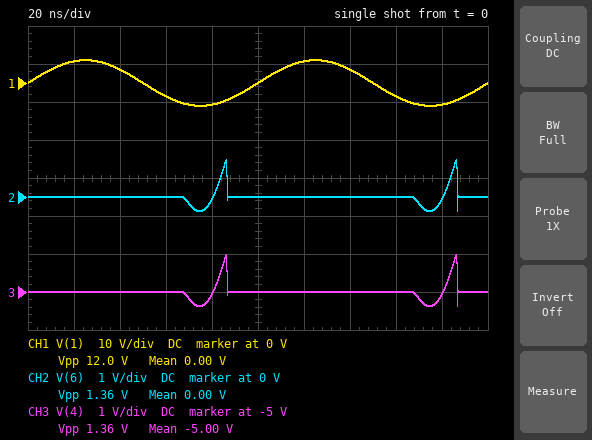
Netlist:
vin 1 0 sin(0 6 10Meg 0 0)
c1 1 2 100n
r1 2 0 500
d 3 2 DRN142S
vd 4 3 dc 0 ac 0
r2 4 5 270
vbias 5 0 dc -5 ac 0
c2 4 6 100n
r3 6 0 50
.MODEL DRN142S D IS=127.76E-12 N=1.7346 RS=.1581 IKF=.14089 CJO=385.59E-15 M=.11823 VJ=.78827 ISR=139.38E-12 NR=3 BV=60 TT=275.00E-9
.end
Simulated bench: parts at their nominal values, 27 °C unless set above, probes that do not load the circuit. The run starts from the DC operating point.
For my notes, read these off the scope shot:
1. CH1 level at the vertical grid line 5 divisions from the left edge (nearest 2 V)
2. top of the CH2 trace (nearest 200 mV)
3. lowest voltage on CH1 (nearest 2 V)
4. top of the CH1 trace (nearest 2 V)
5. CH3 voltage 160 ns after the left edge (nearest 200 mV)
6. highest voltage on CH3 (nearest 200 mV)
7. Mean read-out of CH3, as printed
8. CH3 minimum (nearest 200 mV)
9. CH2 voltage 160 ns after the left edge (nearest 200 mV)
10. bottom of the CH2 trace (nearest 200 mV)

0 V
1.0 V
-6 V
6 V
-5.0 V
-4.0 V
-5.00 V
-5.4 V
0 V
-400 mV
